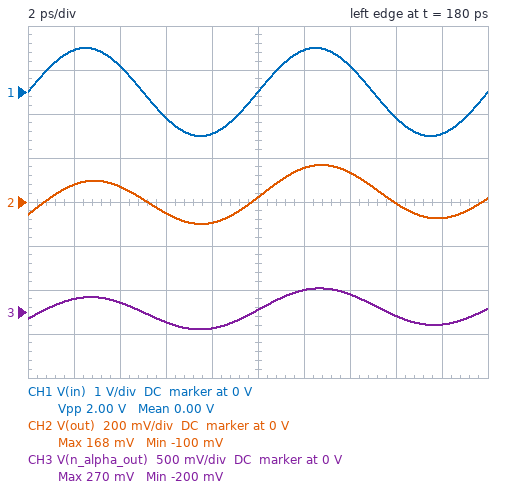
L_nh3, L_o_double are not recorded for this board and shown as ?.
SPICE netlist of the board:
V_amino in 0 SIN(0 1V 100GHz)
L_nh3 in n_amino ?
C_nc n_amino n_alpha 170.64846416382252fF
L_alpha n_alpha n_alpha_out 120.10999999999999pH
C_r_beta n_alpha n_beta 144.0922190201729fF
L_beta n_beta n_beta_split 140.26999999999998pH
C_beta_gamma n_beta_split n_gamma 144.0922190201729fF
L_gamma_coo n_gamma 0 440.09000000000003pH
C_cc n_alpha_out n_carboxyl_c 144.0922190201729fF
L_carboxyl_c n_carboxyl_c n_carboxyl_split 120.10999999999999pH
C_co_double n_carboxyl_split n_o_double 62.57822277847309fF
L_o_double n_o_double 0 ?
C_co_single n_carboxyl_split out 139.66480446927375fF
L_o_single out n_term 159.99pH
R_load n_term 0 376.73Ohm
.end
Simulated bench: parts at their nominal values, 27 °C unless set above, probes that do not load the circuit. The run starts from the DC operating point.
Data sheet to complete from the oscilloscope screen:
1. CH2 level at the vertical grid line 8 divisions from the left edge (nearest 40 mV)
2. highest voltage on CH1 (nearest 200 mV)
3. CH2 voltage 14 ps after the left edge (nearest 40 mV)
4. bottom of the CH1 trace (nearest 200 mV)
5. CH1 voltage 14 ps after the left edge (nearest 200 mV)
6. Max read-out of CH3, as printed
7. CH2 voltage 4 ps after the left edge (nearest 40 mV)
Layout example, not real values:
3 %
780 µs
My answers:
0 V
1.0 V
120 mV
-1.0 V
600 mV
270 mV
80 mV
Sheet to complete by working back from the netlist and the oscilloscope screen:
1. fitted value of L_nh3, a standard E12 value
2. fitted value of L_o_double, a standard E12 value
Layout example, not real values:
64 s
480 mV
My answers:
470 pH
180 pH
